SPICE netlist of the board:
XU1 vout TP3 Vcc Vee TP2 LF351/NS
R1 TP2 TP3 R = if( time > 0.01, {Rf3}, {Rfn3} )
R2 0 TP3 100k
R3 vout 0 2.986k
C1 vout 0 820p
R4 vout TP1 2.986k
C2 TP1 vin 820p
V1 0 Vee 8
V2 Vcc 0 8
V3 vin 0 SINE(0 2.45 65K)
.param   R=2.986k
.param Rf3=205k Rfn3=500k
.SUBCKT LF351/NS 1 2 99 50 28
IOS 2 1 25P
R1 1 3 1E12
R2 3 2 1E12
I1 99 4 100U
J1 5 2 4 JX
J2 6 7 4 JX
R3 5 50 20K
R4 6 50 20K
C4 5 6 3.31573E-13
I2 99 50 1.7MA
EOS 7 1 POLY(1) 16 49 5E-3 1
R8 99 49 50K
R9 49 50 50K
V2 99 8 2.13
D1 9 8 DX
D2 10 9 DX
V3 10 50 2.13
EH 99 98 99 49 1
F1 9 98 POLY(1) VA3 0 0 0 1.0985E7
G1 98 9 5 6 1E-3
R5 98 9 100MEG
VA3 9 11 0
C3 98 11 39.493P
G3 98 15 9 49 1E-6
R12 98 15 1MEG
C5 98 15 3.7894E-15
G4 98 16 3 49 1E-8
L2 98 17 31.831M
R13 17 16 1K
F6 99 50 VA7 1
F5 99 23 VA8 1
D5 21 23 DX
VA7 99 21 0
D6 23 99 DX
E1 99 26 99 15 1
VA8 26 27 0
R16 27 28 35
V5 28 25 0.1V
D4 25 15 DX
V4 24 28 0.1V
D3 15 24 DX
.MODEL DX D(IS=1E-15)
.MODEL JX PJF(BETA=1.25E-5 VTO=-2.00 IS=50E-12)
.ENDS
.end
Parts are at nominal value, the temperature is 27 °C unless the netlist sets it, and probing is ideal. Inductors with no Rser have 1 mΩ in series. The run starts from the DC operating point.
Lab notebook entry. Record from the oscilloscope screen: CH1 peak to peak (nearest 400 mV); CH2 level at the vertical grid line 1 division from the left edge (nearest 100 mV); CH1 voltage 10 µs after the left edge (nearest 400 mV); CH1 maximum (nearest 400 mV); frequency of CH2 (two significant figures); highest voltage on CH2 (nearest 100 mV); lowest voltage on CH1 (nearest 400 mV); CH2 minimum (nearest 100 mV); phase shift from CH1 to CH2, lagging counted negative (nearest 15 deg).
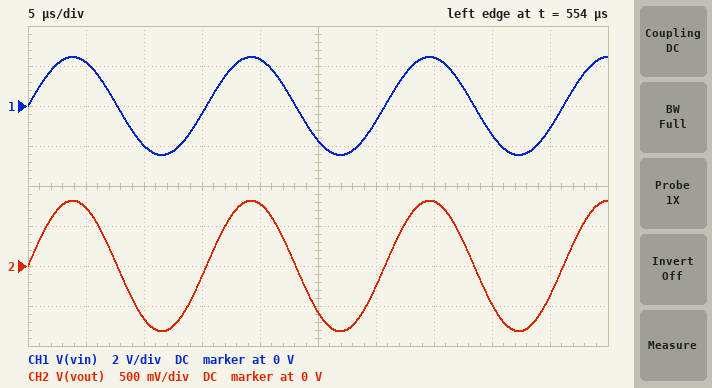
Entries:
4.8 V
700 mV
-2.0 V
2.4 V
65 kHz
800 mV
-2.4 V
-800 mV
0 deg
